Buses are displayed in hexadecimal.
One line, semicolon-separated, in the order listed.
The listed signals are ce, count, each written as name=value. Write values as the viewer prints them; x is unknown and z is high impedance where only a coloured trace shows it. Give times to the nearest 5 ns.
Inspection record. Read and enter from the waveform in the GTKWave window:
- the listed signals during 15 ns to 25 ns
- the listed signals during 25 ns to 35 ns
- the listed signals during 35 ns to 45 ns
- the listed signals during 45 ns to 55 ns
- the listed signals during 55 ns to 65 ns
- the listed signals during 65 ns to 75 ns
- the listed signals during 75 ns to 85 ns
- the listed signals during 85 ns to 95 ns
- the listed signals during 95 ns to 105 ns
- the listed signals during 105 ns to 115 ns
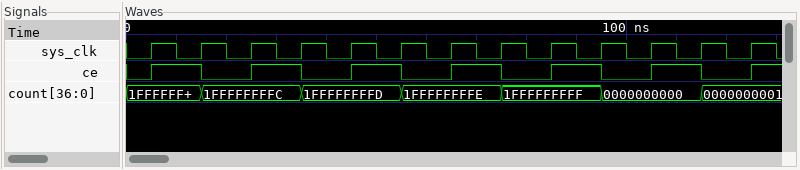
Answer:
ce=0, count=1FFFFFFFFC; ce=1, count=1FFFFFFFFC; ce=0, count=1FFFFFFFFD; ce=1, count=1FFFFFFFFD; ce=0, count=1FFFFFFFFE; ce=1, count=1FFFFFFFFE; ce=0, count=1FFFFFFFFF; ce=1, count=1FFFFFFFFF; ce=0, count=0000000000; ce=1, count=0000000000
